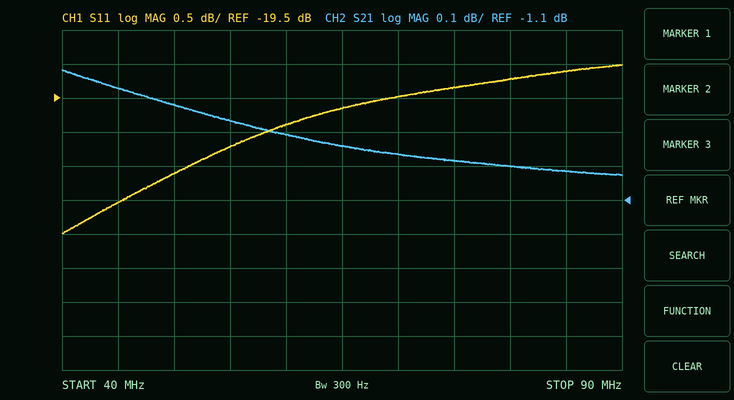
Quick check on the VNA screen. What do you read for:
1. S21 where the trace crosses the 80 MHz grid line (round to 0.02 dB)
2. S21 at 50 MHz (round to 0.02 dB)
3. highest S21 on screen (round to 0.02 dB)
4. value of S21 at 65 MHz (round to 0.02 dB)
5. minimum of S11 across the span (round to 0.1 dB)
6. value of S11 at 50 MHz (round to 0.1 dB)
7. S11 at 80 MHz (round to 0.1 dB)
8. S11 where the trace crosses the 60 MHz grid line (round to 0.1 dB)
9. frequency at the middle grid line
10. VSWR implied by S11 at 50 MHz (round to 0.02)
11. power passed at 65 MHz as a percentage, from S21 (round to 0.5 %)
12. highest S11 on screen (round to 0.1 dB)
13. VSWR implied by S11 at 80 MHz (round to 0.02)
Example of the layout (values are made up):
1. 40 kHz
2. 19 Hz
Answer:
1. -1.00 dB
2. -0.82 dB
3. -0.72 dB
4. -0.94 dB
5. -21.5 dB
6. -20.6 dB
7. -19.2 dB
8. -19.9 dB
9. 65 MHz
10. 1.20
11. 80.5 %
12. -19.0 dB
13. 1.24
